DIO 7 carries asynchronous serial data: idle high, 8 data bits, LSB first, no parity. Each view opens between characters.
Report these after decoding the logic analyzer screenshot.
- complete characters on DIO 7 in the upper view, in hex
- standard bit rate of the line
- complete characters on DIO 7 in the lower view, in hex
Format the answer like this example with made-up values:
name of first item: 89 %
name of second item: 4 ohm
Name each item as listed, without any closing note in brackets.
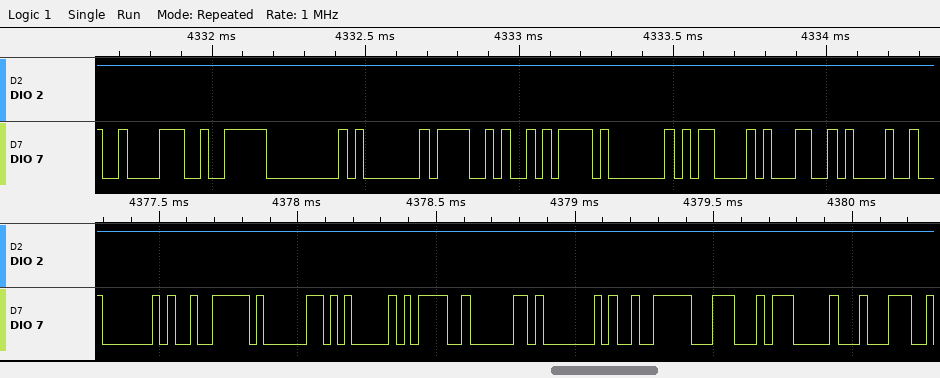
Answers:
complete characters on DIO 7 in the upper view, in hex: C2, F2, 00, 01, 4F, EA, 01, 0D, 31, 21
standard bit rate of the line: 38400 baud
complete characters on DIO 7 in the lower view, in hex: 40, F2, 81, 05, 3D, 60, 40, F2, 1C, 07, C4
